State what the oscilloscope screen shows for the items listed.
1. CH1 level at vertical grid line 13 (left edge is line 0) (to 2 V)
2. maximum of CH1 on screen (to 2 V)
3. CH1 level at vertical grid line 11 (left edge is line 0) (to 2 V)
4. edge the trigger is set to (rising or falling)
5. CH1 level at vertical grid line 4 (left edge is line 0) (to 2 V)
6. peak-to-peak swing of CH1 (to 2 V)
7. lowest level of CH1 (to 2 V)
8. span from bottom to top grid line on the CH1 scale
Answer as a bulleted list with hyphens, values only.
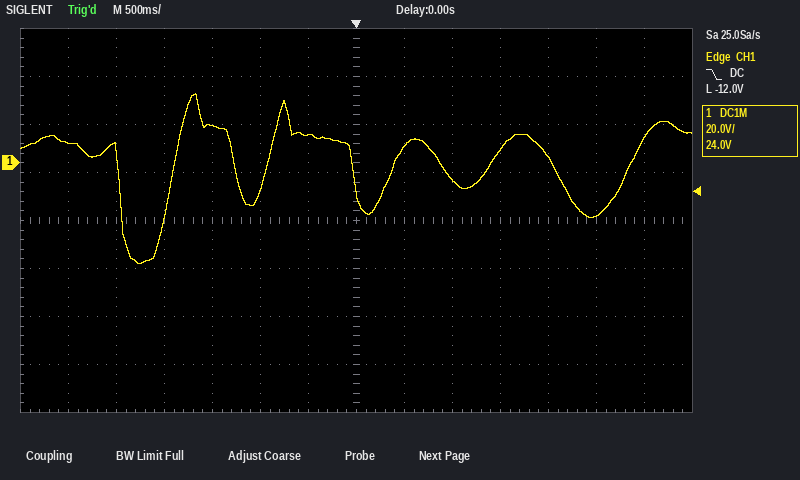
- 10 V
- 28 V
- 2 V
- falling
- 16 V
- 70 V
- -42 V
- 160 V
